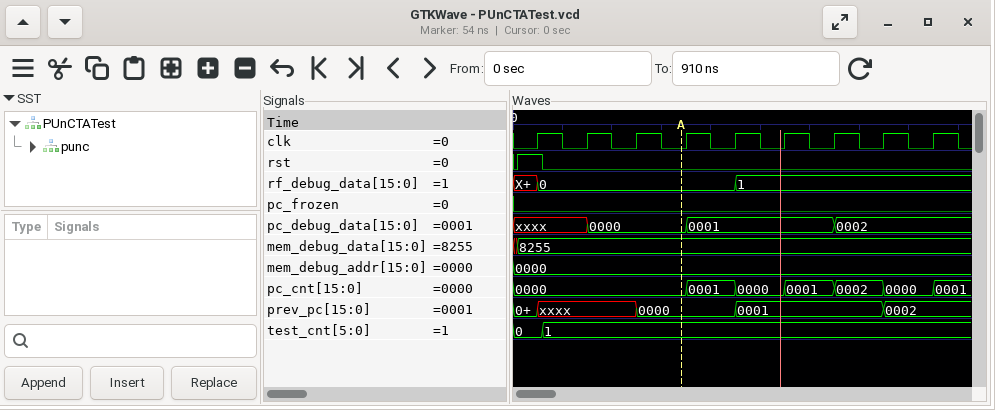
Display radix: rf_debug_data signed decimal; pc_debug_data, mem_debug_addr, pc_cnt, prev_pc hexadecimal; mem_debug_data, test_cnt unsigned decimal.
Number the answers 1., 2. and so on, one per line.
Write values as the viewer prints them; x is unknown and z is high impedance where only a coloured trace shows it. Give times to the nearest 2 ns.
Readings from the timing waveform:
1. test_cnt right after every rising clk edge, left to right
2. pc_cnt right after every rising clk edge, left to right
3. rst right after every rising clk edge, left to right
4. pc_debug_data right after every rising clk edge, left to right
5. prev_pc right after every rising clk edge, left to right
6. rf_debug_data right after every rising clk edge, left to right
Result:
1. 0, 1, 1, 1, 1, 1, 1, 1, 1
2. 0000, 0000, 0000, 0001, 0000, 0001, 0002, 0000, 0001
3. 1 0 0 0 0 0 0 0 0
4. xxxx, 0000, 0000, 0001, 0001, 0001, 0002, 0002, 0002
5. xxxx, xxxx, 0000, 0000, 0001, 0001, 0001, 0002, 0002
6. 0, 0, 0, 0, 1, 1, 1, 1, 1
